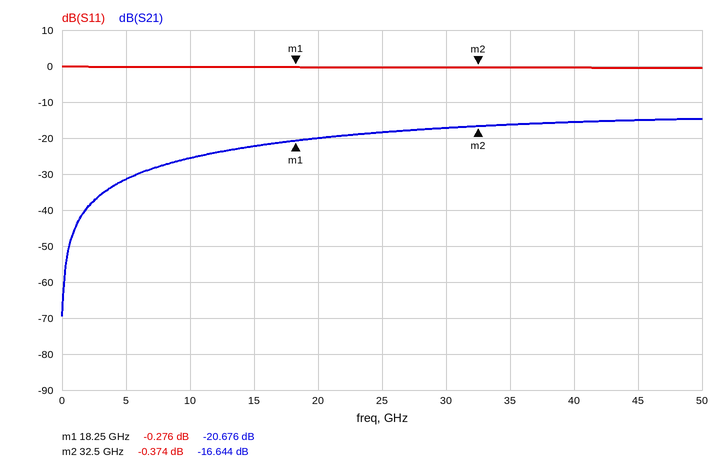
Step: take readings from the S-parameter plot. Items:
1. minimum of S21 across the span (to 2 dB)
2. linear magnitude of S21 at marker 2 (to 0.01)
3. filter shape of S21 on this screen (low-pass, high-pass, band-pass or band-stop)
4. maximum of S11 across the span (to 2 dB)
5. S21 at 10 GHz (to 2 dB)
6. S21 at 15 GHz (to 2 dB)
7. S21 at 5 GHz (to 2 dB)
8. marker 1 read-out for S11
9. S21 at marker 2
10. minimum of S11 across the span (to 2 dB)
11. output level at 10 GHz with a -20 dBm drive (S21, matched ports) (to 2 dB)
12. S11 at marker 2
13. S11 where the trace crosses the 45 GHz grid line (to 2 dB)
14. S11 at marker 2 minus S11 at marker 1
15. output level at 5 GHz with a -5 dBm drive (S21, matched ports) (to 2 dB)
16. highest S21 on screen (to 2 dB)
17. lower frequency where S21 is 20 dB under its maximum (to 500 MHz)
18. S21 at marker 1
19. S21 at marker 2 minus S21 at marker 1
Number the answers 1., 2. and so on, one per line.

1. -70 dB
2. 0.15
3. high-pass
4. 0 dB
5. -26 dB
6. -22 dB
7. -32 dB
8. -0.276 dB
9. -16.644 dB
10. 0 dB
11. -46 dBm
12. -0.374 dB
13. 0 dB
14. -0.098 dB
15. -36 dBm
16. -14 dB
17. 3.5 GHz
18. -20.676 dB
19. 4.032 dB
